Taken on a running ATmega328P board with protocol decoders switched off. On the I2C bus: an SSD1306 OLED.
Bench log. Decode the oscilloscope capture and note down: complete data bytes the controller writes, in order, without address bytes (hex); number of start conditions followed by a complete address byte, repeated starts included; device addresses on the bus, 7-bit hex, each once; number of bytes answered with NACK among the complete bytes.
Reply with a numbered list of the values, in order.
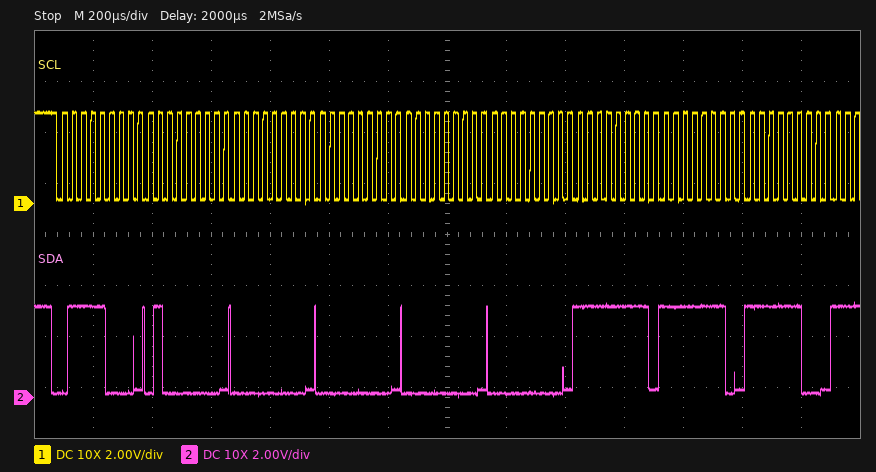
1. 40 00 00 00 00 FF FE FC
2. 1
3. 0x3C
4. 0
